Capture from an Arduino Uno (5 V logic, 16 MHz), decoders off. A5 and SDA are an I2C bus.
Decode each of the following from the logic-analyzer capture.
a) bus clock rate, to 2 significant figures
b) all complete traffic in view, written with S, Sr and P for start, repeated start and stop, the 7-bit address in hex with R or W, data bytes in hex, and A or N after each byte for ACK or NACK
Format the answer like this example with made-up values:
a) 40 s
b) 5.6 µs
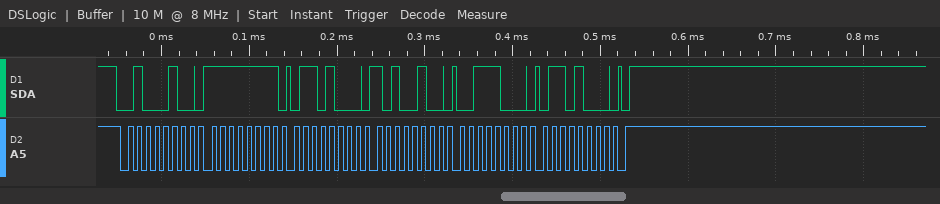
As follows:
a) 100 kHz
b) S 22W A FF A 68 A A4 A 38 A 68 A P
